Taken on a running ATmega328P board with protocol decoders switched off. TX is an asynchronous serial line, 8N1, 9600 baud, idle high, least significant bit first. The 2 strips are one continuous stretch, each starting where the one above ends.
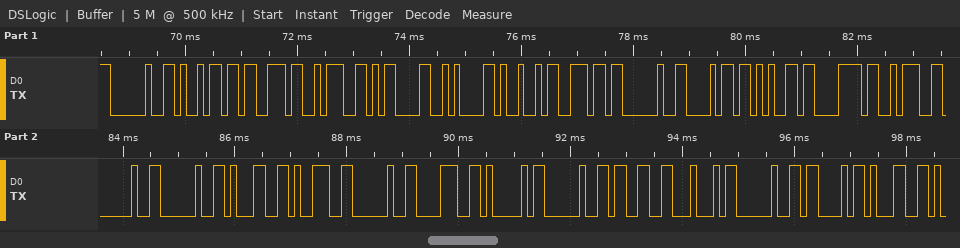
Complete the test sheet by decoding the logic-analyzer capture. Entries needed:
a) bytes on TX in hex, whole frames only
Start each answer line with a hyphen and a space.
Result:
- 20 69 73 3A 0D 0A 49 6E 20 68 65 78 3A 20 20 31 39 20 38 41 20 33 44 20 43 31
